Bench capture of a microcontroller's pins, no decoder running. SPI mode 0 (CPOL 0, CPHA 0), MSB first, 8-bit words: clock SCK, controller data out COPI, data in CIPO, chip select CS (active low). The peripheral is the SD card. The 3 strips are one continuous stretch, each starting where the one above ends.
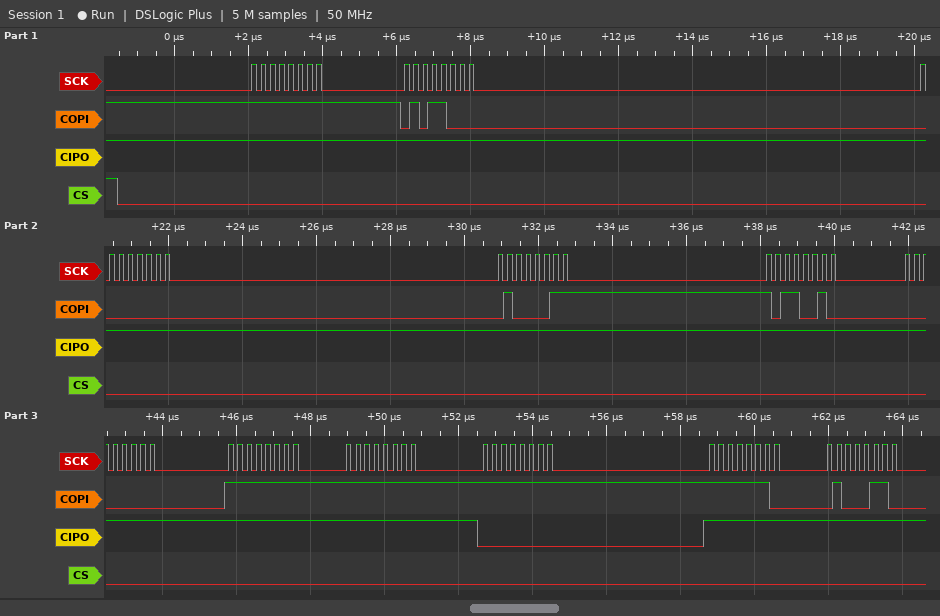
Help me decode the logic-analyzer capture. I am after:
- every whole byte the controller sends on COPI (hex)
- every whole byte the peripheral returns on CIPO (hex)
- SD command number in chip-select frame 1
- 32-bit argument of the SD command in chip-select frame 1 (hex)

FF 58 00 43 B2 00 FF FF FF FE 46
FF FF FF FF FF FF FF FF 00 FF FF
CMD24
0x0043B200
